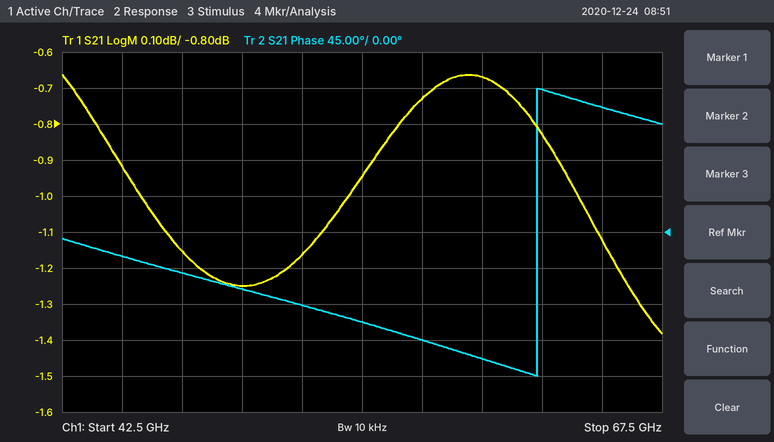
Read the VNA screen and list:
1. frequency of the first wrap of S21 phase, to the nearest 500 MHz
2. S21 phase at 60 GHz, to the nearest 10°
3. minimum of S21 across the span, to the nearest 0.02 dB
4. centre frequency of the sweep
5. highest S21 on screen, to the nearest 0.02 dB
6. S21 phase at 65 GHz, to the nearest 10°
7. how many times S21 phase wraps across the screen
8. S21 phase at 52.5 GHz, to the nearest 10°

62.5 GHz
-160°
-1.38 dB
55 GHz
-0.66 dB
160°
1
-90°
